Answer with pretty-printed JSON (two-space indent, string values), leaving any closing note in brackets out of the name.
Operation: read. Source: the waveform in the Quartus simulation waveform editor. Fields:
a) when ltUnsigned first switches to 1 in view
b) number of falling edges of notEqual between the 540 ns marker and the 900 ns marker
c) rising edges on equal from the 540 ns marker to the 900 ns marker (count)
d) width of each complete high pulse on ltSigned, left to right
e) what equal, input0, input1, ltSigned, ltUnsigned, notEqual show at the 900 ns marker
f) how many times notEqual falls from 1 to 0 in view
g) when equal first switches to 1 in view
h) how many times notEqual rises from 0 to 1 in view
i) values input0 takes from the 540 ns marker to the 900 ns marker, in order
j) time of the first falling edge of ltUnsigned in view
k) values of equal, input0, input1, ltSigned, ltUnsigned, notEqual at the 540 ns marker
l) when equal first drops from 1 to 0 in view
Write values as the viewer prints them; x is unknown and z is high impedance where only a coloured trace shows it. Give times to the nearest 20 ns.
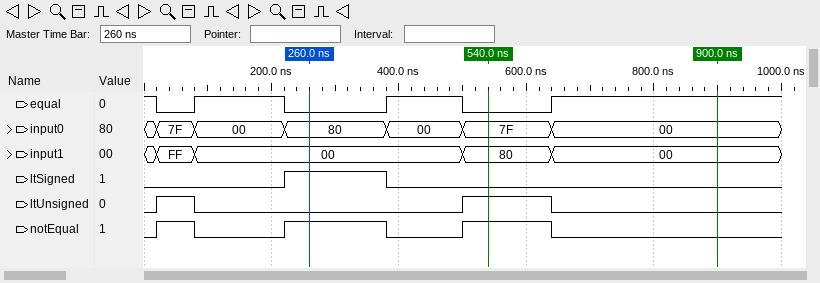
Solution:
{
  "when ltUnsigned first switches to 1 in view": "20 ns",
  "number of falling edges of notEqual between the 540 ns marker and the 900 ns marker": "1",
  "rising edges on equal from the 540 ns marker to the 900 ns marker": "1",
  "width of each complete high pulse on ltSigned, left to right": "160 ns",
  "what equal, input0, input1, ltSigned, ltUnsigned, notEqual show at the 900 ns marker": "equal=1, input0=00, input1=00, ltSigned=0, ltUnsigned=0, notEqual=0",
  "how many times notEqual falls from 1 to 0 in view": "3",
  "when equal first switches to 1 in view": "80 ns",
  "how many times notEqual rises from 0 to 1 in view": "3",
  "values input0 takes from the 540 ns marker to the 900 ns marker, in order": "7F, 00",
  "time of the first falling edge of ltUnsigned in view": "80 ns",
  "values of equal, input0, input1, ltSigned, ltUnsigned, notEqual at the 540 ns marker": "equal=0, input0=7F, input1=80, ltSigned=0, ltUnsigned=1, notEqual=1",
  "when equal first drops from 1 to 0 in view": "20 ns"
}
